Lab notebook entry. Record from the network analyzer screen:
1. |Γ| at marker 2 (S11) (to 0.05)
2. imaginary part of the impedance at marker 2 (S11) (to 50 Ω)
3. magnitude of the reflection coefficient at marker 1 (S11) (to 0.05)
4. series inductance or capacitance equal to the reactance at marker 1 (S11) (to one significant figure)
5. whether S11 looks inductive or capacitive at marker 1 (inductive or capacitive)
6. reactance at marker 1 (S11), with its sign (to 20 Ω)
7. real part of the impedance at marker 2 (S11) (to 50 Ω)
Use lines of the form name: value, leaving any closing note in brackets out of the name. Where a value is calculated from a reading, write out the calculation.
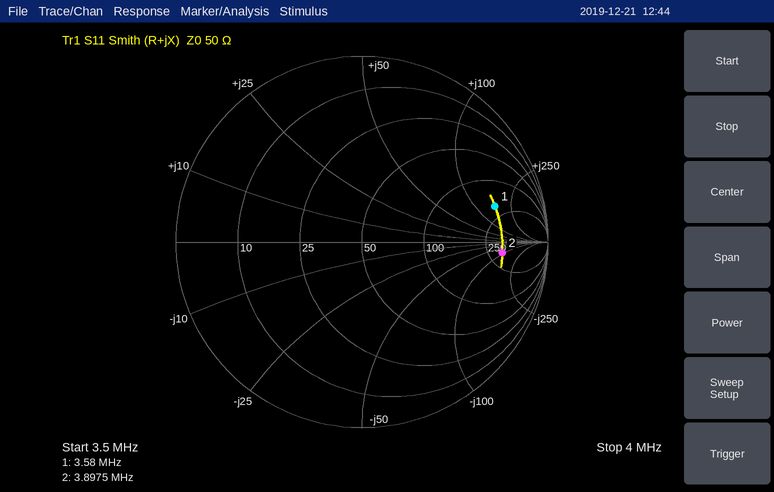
|Γ| at marker 2 (S11): 0.75
imaginary part of the impedance at marker 2 (S11): -100 Ω
magnitude of the reflection coefficient at marker 1 (S11): 0.75
series inductance or capacitance equal to the reactance at marker 1 (S11): L = 160 Ω/(2π × 3.58 MHz) ≈ 7 µH
whether S11 looks inductive or capacitive at marker 1: inductive
reactance at marker 1 (S11), with its sign: +160 Ω
real part of the impedance at marker 2 (S11): 350 Ω
